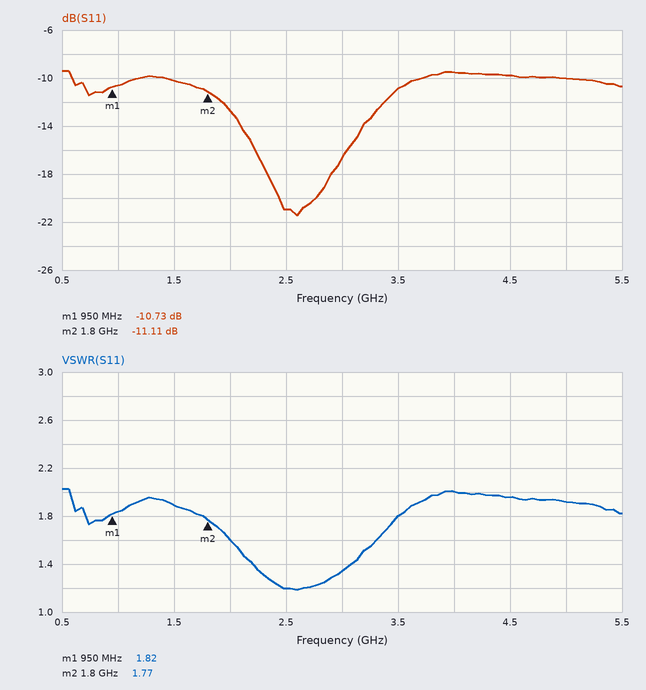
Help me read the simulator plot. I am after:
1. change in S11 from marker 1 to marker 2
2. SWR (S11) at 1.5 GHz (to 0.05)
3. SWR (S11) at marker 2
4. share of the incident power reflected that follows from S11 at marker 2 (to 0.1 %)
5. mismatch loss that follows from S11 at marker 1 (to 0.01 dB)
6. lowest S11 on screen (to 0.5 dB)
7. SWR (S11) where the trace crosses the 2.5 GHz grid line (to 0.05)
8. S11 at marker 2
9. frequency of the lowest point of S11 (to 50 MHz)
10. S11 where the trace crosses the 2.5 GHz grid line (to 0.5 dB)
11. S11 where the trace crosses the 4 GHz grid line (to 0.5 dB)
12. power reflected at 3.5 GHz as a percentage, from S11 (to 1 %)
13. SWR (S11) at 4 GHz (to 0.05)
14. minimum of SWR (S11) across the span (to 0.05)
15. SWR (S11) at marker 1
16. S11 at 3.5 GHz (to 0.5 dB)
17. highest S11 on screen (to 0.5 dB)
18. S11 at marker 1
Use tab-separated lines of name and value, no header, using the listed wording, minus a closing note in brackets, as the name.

change in S11 from marker 1 to marker 2	-0.38 dB
SWR (S11) at 1.5 GHz	1.90
SWR (S11) at marker 2	1.77
share of the incident power reflected that follows from S11 at marker 2	7.7 %
mismatch loss that follows from S11 at marker 1	0.38 dB
lowest S11 on screen	-21.5 dB
SWR (S11) where the trace crosses the 2.5 GHz grid line	1.20
S11 at marker 2	-11.11 dB
frequency of the lowest point of S11	2.60 GHz
S11 where the trace crosses the 2.5 GHz grid line	-21.0 dB
S11 where the trace crosses the 4 GHz grid line	-9.5 dB
power reflected at 3.5 GHz as a percentage, from S11	8 %
SWR (S11) at 4 GHz	2.00
minimum of SWR (S11) across the span	1.20
SWR (S11) at marker 1	1.82
S11 at 3.5 GHz	-11.0 dB
highest S11 on screen	-9.5 dB
S11 at marker 1	-10.73 dB
